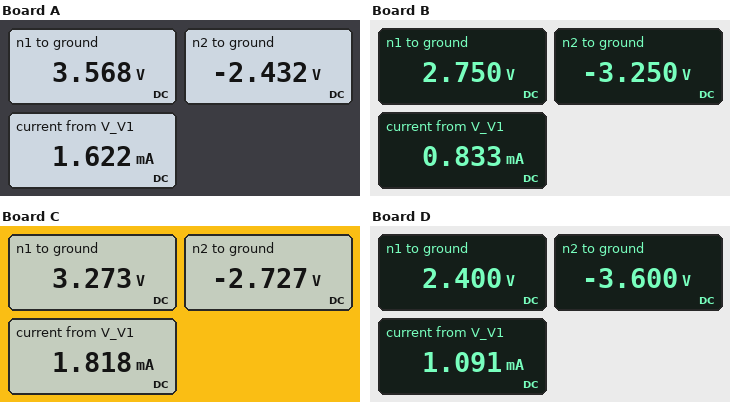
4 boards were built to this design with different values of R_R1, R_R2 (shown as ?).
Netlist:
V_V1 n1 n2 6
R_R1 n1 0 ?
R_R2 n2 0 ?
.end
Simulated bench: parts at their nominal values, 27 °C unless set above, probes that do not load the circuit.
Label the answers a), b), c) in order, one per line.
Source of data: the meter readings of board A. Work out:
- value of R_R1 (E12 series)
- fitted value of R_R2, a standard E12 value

a) 2.2 kΩ
b) 1.5 kΩ
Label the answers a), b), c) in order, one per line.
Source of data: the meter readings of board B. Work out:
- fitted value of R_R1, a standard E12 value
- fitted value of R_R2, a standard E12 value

a) 3.3 kΩ
b) 3.9 kΩ
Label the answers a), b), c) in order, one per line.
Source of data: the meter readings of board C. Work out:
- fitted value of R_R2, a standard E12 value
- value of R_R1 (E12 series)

a) 1.5 kΩ
b) 1.8 kΩ
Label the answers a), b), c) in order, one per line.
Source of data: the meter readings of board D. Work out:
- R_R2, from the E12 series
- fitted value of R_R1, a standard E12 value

a) 3.3 kΩ
b) 2.2 kΩ
